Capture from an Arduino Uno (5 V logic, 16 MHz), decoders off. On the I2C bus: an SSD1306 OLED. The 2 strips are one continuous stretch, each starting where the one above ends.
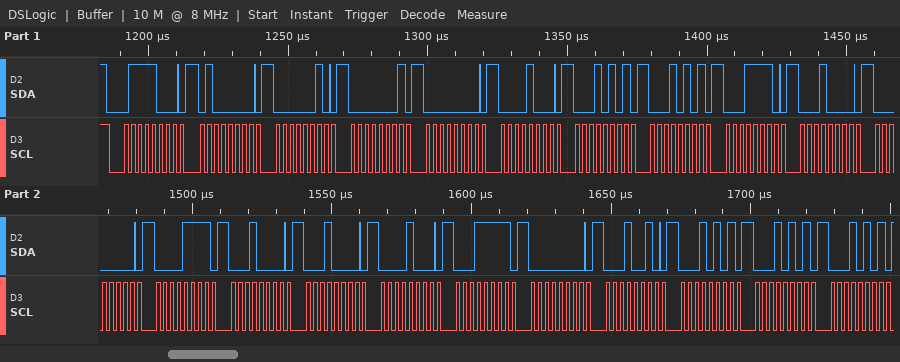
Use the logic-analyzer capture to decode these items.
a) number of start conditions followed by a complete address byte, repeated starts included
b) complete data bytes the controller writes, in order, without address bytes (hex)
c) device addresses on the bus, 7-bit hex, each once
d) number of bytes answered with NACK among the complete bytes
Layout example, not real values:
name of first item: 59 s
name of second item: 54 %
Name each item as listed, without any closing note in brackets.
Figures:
number of start conditions followed by a complete address byte, repeated starts included: 1
complete data bytes the controller writes, in order, without address bytes: 40 02 01 00 08 15 15 1E 10 00 0F 10 10 08 1F 00 12 15 15 15
device addresses on the bus, 7-bit hex, each once: 0x3C
number of bytes answered with NACK among the complete bytes: 0
